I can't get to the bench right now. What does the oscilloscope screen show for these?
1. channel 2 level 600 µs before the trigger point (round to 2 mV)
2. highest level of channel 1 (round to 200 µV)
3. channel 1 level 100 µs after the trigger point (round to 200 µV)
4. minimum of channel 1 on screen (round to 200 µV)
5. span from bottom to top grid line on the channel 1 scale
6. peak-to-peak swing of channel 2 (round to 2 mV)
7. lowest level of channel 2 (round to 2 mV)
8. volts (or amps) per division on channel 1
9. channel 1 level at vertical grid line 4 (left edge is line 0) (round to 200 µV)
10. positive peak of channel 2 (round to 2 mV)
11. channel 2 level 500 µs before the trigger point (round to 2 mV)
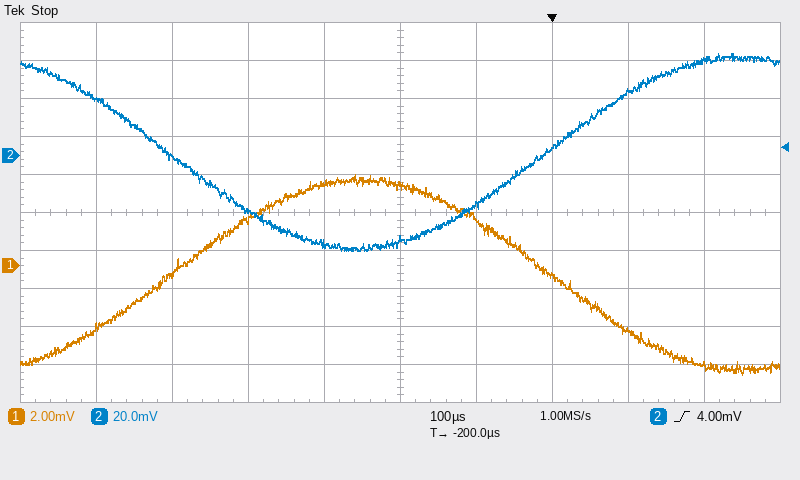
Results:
30 mV
4.8 mV
-3.4 mV
-5.8 mV
20 mV
104 mV
-50 mV
2 mV
4.4 mV
54 mV
0 mV
